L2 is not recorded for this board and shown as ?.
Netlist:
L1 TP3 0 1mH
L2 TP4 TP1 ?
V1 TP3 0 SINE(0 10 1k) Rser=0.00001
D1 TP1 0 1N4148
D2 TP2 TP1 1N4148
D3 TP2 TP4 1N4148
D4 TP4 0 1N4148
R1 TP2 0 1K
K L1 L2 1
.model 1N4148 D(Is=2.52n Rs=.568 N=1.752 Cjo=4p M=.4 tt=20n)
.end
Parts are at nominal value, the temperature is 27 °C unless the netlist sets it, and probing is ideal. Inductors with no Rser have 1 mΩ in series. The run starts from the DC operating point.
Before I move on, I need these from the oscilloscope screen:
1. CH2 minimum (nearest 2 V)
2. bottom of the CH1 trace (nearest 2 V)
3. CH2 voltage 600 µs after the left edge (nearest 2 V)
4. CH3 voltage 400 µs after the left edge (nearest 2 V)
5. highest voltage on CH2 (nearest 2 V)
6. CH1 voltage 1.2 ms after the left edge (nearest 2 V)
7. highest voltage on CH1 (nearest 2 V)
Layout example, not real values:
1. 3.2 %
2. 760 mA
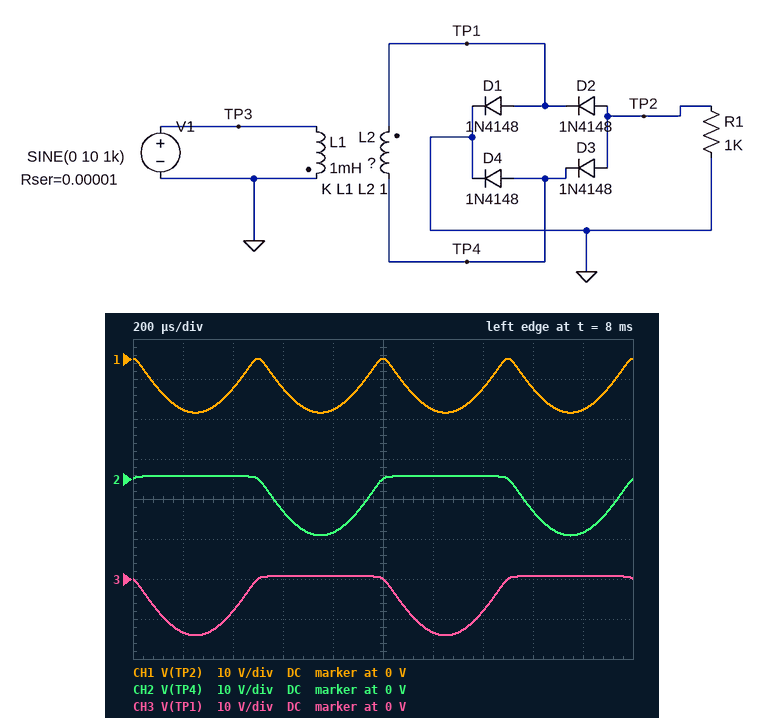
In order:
1. -14 V
2. -14 V
3. -8 V
4. -8 V
5. 0 V
6. -12 V
7. 0 V
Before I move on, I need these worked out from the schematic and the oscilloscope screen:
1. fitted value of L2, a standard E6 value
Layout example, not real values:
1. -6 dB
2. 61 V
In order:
1. 2.2 mH
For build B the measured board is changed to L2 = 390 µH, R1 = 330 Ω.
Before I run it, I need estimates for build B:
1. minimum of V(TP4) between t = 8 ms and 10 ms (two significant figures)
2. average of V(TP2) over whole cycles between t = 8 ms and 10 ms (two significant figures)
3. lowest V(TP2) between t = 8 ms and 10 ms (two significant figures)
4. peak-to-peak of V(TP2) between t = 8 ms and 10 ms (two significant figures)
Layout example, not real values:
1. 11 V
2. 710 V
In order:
1. -5.5 V
2. -2.7 V
3. -4.8 V
4. 4.8 V
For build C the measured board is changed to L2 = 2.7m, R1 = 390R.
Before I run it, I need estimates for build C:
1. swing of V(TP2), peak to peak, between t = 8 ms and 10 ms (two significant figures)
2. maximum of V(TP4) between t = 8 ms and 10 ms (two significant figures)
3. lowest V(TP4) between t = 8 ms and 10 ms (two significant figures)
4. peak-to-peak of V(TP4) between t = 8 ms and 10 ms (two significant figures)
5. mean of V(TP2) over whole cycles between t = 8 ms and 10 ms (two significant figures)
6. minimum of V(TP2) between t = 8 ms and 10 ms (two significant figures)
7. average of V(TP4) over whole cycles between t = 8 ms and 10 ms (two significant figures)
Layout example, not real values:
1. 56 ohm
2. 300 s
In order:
1. 15 V
2. 770 mV
3. -16 V
4. 16 V
5. -9.0 V
6. -15 V
7. -4.5 V
